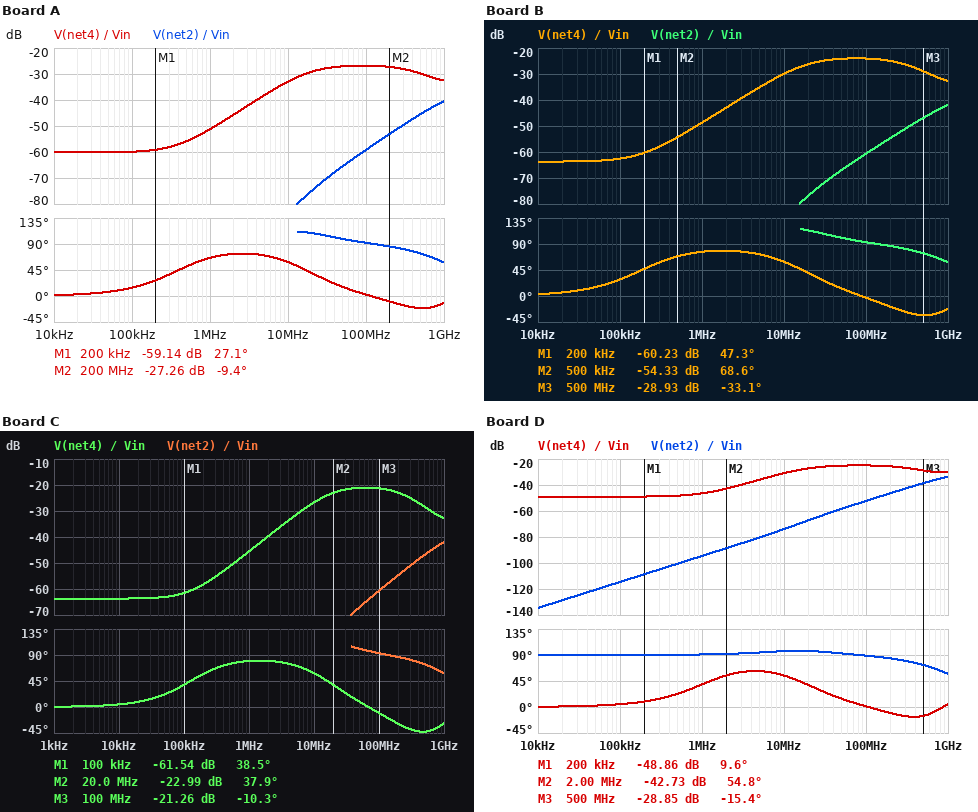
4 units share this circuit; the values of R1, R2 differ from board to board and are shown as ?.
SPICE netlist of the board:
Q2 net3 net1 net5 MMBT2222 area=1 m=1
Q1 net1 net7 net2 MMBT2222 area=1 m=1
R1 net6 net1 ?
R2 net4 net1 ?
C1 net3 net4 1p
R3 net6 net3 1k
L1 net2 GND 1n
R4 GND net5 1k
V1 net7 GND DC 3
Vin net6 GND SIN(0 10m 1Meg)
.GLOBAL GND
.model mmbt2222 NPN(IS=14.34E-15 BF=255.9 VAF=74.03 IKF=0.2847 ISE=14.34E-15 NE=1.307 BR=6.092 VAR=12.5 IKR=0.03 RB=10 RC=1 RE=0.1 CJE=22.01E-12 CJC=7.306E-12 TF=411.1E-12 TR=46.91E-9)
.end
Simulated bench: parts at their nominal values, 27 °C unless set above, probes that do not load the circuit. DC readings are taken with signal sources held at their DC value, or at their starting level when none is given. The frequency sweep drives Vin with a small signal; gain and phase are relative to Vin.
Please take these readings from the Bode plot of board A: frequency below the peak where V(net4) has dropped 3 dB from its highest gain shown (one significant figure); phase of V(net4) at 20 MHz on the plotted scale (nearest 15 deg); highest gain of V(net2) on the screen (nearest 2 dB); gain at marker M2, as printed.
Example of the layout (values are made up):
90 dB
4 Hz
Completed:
20 MHz
45 deg
-40 dB
-27.26 dB
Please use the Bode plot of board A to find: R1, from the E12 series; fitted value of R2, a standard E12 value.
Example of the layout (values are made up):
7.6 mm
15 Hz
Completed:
1.2 kΩ
390 Ω
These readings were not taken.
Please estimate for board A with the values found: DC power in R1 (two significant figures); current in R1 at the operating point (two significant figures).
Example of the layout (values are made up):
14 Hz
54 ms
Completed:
1.6 µW
36 µA
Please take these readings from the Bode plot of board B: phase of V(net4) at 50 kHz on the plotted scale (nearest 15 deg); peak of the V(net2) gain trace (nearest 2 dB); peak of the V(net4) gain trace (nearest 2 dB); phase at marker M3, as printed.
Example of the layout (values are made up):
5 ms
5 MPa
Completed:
15 deg
-42 dB
-24 dB
-33.1 deg
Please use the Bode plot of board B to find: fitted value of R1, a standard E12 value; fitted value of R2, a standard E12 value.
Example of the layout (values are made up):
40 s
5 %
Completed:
1.8 kΩ
560 Ω
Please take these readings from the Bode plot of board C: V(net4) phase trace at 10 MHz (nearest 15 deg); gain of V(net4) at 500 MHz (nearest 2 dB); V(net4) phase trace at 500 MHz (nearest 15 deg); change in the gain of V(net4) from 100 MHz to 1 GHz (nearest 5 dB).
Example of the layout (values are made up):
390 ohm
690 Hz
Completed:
60 deg
-28 dB
-45 deg
-10 dB
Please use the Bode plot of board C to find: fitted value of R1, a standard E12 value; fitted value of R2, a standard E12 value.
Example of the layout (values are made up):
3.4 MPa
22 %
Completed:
1.8 kΩ
820 Ω
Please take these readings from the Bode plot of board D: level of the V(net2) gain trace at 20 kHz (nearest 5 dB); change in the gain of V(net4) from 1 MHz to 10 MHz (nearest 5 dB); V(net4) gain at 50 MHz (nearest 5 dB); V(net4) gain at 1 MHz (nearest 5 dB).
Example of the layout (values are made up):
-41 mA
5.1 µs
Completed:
-130 dB
15 dB
-25 dB
-45 dB
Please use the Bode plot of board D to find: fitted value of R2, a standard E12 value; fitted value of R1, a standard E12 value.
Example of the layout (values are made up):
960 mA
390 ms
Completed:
470 Ω
330 Ω
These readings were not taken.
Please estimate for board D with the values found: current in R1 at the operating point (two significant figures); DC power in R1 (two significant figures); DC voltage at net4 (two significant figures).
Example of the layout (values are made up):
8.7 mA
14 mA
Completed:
130 µA
5.7 µW
43 mV
